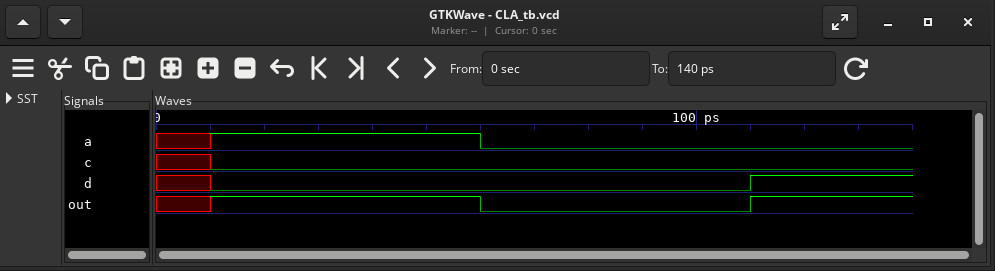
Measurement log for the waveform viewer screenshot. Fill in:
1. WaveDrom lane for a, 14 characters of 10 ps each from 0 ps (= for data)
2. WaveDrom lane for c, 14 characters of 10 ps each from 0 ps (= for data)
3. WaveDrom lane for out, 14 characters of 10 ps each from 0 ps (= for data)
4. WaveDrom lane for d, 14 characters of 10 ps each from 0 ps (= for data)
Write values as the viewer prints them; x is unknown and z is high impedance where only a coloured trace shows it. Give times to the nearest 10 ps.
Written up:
{name: 'a', wave: 'x1....0.......'}
{name: 'c', wave: 'x0............'}
{name: 'out', wave: 'x1....0....1..'}
{name: 'd', wave: 'x0.........1..'}
